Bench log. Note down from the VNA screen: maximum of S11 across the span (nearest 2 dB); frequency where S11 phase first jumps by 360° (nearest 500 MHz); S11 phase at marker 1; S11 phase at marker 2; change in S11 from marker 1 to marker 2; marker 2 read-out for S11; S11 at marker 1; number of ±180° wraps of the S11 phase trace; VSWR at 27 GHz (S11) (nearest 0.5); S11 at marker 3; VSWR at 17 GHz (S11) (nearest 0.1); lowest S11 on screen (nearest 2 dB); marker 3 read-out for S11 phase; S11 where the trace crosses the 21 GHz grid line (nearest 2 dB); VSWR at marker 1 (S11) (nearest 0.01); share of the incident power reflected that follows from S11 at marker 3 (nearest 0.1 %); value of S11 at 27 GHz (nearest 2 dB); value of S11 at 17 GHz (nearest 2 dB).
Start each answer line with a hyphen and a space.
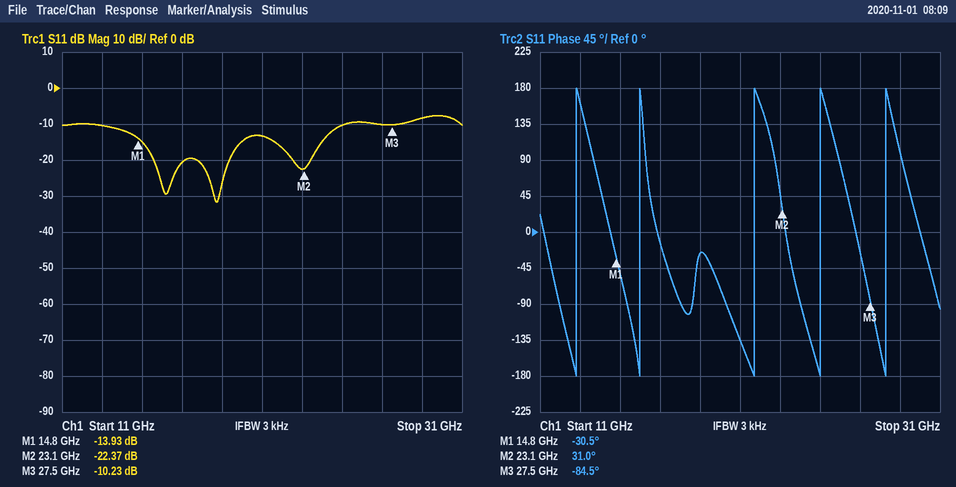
- -8 dB
- 13.0 GHz
- -30.5°
- 31.0°
- -8.44 dB
- -22.37 dB
- -13.93 dB
- 5
- 2.0
- -10.23 dB
- 1.2
- -32 dB
- -84.5°
- -14 dB
- 1.50
- 9.5 %
- -10 dB
- -20 dB
